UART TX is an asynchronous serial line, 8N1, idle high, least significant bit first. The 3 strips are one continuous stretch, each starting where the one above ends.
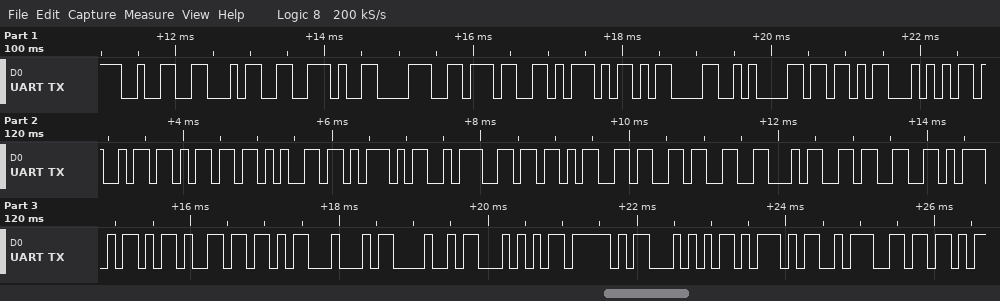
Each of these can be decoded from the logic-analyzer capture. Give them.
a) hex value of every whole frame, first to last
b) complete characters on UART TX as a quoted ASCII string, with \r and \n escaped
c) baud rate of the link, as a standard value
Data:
32 34 2E 38 37 5D 0D 0A 5B 54 69 6D 65 5D 3A 5B 36 33 34 33 5D 2D 5B 44 48 54 5F 54 5D 3A 5B
"24.87]\r\n[Time]:[6343]-[DHT_T]:["
9600 baud
